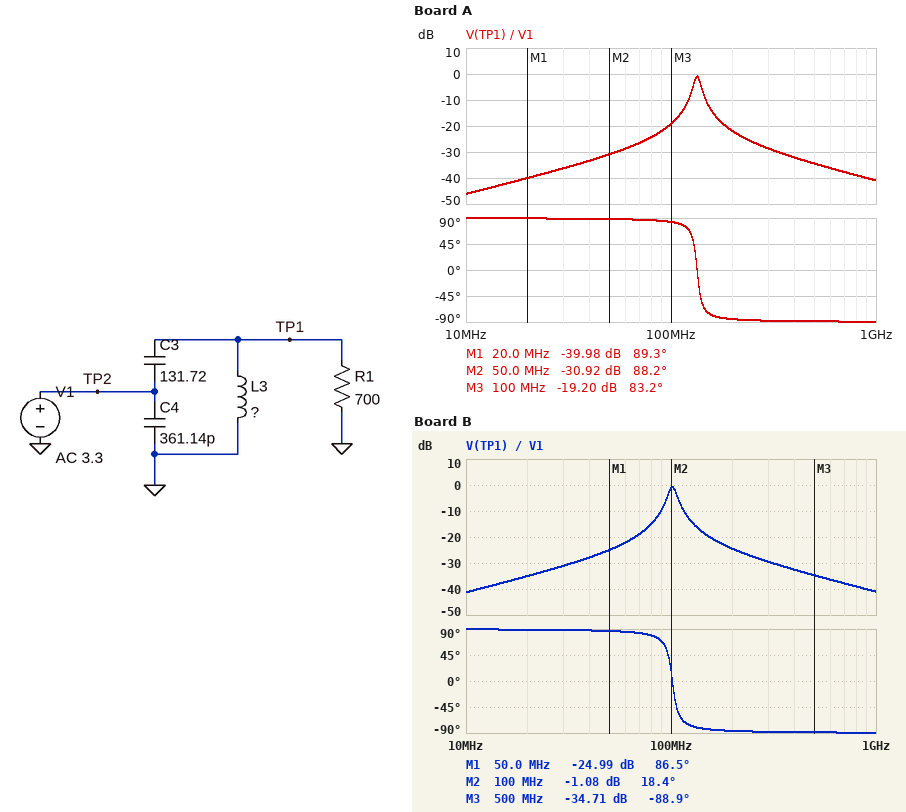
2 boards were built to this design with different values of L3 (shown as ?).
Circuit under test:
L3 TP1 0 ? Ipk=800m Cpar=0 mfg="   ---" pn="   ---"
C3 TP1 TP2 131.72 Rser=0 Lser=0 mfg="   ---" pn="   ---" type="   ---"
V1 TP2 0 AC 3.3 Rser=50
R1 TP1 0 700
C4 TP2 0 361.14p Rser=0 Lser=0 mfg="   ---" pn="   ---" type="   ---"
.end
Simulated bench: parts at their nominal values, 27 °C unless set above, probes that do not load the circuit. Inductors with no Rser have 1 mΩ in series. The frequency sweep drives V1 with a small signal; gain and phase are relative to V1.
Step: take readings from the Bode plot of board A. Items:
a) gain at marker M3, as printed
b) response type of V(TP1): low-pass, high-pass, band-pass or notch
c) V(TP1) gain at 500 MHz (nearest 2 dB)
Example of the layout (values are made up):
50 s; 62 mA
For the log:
-19.20 dB; band-pass; -34 dB
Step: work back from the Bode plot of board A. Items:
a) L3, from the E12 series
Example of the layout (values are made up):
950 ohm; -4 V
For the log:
3.9 nH
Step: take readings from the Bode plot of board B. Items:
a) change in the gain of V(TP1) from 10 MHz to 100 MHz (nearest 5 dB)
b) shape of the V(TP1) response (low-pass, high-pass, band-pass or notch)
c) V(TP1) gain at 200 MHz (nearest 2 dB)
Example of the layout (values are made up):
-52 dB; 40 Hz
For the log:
40 dB; band-pass; -24 dB
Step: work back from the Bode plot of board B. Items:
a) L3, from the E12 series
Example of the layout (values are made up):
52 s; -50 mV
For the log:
6.8 nH
